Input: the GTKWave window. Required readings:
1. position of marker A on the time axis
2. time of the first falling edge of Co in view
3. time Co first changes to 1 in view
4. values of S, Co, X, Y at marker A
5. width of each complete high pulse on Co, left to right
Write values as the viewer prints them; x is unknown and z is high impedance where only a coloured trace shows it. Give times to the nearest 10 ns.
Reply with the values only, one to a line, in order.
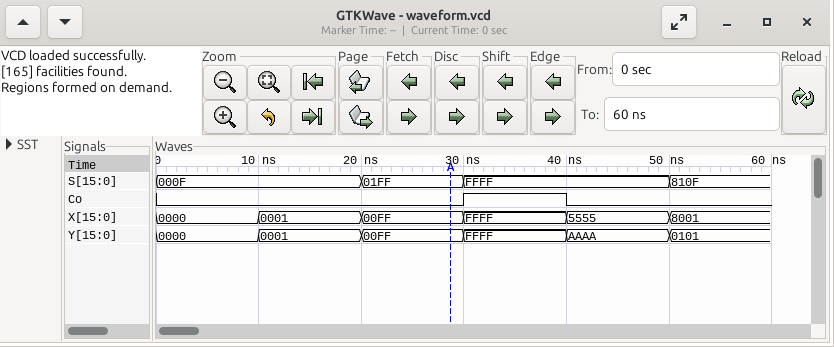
30 ns
40 ns
30 ns
S=01FF, Co=0, X=00FF, Y=00FF
10 ns
